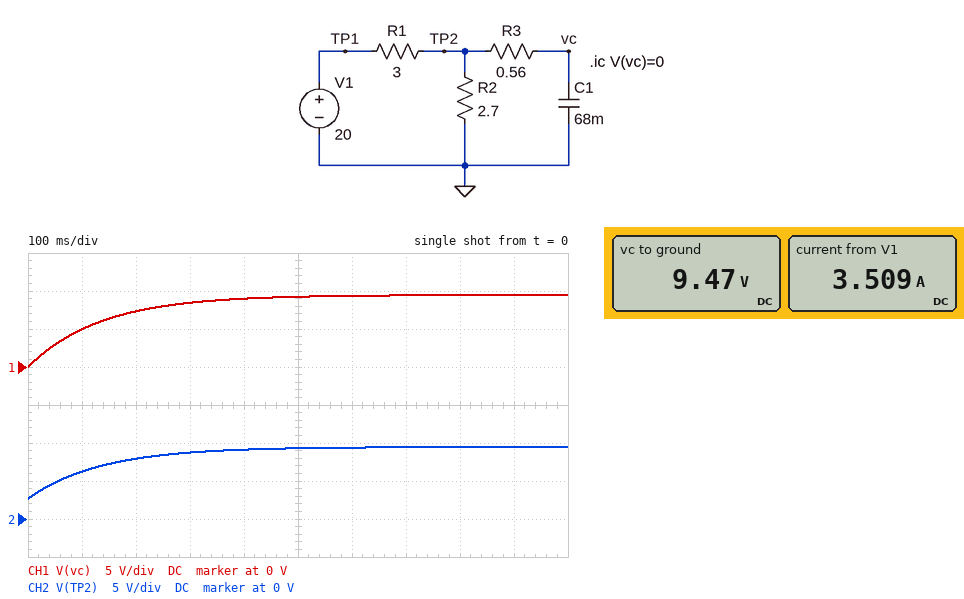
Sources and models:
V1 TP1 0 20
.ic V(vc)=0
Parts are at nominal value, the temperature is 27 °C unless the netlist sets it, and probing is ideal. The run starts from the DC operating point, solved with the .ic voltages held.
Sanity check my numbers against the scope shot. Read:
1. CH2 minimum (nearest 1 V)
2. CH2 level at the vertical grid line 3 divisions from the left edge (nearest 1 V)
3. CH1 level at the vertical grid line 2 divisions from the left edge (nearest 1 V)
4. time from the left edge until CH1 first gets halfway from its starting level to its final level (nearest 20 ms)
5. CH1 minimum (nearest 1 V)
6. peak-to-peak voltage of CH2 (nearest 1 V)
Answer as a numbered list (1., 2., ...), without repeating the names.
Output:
1. 3 V
2. 9 V
3. 7 V
4. 100 ms
5. 0 V
6. 7 V
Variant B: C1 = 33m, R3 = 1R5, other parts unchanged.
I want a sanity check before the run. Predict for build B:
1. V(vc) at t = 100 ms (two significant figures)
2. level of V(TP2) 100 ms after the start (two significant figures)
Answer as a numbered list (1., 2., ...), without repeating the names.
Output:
1. 6.1 V
2. 7.8 V
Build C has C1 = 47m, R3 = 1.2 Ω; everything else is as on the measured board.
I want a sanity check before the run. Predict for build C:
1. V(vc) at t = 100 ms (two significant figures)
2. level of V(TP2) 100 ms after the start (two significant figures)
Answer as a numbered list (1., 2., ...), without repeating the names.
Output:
1. 5.3 V
2. 7.2 V
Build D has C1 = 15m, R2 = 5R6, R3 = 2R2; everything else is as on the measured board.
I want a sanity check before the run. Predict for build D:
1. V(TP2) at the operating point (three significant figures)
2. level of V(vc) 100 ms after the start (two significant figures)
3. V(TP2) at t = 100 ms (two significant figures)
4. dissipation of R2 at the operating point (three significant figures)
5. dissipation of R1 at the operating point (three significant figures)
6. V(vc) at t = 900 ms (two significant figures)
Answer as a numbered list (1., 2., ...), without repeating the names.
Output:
1. 13.0 V
2. 10 V
3. 12 V
4. 30.3 W
5. 16.2 W
6. 13 V
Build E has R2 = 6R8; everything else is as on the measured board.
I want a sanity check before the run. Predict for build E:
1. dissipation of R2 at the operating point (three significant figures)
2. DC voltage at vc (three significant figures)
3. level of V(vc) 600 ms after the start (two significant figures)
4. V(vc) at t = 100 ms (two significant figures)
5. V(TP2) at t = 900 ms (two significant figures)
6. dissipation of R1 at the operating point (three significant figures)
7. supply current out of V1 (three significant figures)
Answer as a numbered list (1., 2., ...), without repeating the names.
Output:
1. 28.3 W
2. 13.9 V
3. 13 V
4. 5.9 V
5. 14 V
6. 12.5 W
7. 2.04 A
